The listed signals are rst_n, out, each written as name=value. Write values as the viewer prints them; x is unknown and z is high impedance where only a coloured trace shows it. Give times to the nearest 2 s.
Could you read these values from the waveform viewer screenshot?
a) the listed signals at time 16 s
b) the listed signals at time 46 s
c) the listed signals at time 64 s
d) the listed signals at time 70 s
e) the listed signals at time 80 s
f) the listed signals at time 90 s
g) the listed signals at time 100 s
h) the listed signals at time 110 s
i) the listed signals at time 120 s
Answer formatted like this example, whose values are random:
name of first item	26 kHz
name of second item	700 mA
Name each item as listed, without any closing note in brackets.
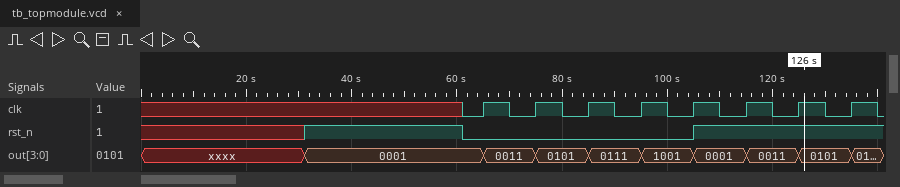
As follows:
the listed signals at time 16 s	rst_n=x, out=xxxx
the listed signals at time 46 s	rst_n=1, out=0001
the listed signals at time 64 s	rst_n=0, out=0001
the listed signals at time 70 s	rst_n=0, out=0011
the listed signals at time 80 s	rst_n=0, out=0101
the listed signals at time 90 s	rst_n=0, out=0111
the listed signals at time 100 s	rst_n=0, out=1001
the listed signals at time 110 s	rst_n=1, out=0001
the listed signals at time 120 s	rst_n=1, out=0011
